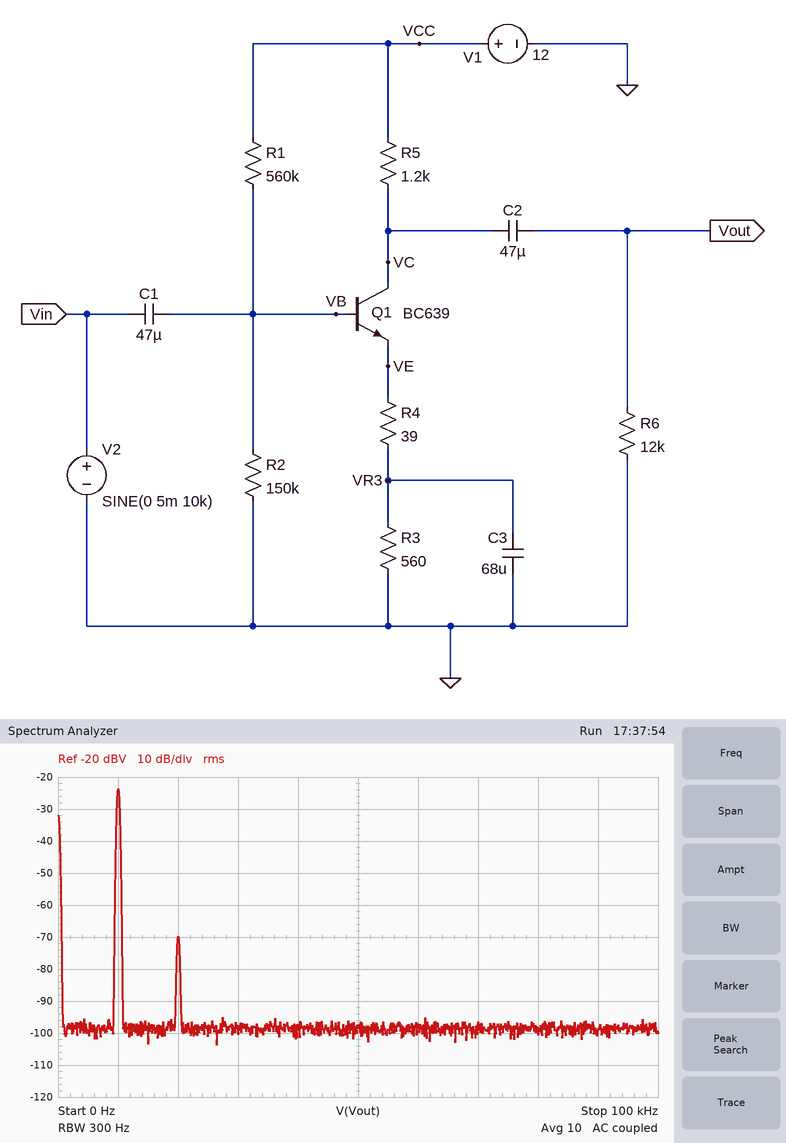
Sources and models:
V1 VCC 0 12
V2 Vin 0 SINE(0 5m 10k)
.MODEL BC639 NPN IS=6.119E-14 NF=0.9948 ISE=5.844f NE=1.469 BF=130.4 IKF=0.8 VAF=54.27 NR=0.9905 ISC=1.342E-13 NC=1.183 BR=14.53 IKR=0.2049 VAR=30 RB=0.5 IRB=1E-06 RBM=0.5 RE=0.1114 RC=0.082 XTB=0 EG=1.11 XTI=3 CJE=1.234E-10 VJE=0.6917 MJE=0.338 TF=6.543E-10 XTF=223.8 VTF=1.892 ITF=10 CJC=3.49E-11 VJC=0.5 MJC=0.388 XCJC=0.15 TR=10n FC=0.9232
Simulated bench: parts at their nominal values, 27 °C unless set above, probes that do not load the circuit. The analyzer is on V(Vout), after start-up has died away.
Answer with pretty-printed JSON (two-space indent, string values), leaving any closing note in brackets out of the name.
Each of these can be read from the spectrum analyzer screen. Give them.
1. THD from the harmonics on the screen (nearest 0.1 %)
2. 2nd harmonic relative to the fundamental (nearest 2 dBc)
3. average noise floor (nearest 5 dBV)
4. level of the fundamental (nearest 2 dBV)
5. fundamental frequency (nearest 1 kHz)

{
  "THD from the harmonics on the screen": "0.5 %",
  "2nd harmonic relative to the fundamental": "-46 dBc",
  "average noise floor": "-100 dBV",
  "level of the fundamental": "-24 dBV",
  "fundamental frequency": "10 kHz"
}
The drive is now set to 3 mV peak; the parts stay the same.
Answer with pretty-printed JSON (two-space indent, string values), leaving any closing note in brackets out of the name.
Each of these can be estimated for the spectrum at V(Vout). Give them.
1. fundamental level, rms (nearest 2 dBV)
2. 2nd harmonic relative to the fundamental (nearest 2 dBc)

{
  "fundamental level, rms": "-28 dBV",
  "2nd harmonic relative to the fundamental": "-50 dBc"
}
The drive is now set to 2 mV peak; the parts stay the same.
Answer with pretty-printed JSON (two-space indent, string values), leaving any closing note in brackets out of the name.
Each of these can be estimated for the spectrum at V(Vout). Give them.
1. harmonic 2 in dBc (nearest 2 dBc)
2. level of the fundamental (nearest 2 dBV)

{
  "harmonic 2 in dBc": "-54 dBc",
  "level of the fundamental": "-32 dBV"
}
